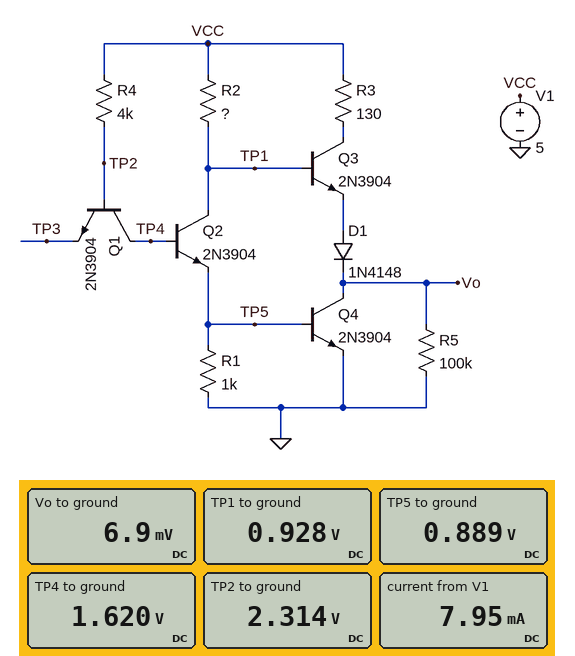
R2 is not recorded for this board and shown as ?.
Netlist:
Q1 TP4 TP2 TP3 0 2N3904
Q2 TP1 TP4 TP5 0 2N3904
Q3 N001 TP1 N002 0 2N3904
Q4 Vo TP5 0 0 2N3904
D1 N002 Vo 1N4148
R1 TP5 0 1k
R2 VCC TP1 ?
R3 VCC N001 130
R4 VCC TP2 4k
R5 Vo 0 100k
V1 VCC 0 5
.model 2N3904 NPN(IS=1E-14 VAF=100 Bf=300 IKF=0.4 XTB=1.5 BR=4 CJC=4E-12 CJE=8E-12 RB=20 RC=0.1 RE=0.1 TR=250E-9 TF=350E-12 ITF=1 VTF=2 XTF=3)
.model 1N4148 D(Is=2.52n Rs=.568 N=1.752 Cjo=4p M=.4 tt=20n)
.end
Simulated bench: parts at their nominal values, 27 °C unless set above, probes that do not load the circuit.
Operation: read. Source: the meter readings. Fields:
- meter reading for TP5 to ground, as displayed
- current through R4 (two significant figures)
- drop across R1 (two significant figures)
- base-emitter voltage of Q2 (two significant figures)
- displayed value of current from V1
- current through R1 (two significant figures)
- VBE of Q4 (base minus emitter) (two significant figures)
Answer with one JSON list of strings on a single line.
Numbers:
["0.889 V", "670 µA", "890 mV", "730 mV", "7.95 mA", "890 µA", "890 mV"]
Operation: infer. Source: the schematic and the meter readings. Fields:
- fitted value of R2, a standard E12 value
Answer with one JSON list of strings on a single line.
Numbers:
["560 Ω"]
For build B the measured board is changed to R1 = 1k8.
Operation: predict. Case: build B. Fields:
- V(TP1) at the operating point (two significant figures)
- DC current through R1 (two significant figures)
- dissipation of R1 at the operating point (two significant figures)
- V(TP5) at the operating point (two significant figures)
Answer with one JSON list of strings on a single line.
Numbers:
["940 mV", "500 µA", "450 µW", "900 mV"]
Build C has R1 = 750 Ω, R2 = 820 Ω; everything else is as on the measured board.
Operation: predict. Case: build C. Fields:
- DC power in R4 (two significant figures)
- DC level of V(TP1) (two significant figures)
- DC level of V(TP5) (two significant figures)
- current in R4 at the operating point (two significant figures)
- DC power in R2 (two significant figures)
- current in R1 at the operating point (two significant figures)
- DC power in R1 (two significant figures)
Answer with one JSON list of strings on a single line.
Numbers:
["1.9 mW", "860 mV", "830 mV", "690 µA", "21 mW", "1.1 mA", "920 µW"]
